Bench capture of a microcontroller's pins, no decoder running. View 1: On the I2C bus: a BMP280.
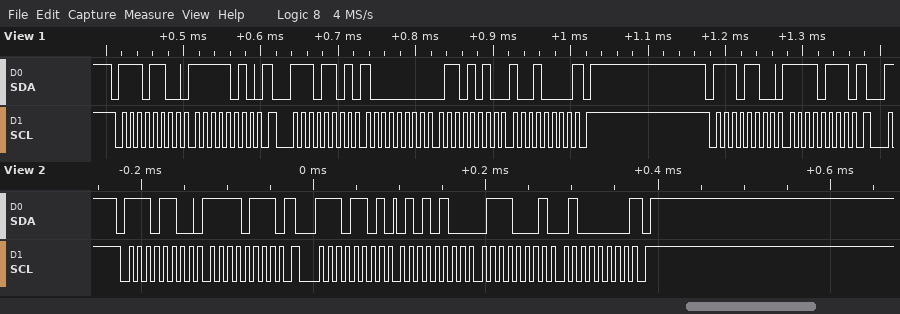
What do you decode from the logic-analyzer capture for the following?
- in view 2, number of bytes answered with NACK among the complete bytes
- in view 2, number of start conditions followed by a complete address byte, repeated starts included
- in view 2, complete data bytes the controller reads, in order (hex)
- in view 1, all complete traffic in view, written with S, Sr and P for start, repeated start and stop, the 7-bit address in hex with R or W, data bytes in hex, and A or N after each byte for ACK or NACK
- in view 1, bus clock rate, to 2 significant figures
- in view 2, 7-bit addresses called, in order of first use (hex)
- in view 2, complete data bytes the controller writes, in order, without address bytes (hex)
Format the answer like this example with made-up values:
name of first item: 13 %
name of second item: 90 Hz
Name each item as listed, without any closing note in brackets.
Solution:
in view 2, number of bytes answered with NACK among the complete bytes: 1
in view 2, number of start conditions followed by a complete address byte, repeated starts included: 2
in view 2, complete data bytes the controller reads, in order: 54 71 40
in view 1, all complete traffic in view, written with S, Sr and P for start, repeated start and stop, the 7-bit address in hex with R or W, data bytes in hex, and A or N after each byte for ACK or NACK: S 76W A FA A Sr 76R A 80 A 6A A 90 N P S 76W A F7 A
in view 1, bus clock rate, to 2 significant figures: 100 kHz
in view 2, 7-bit addresses called, in order of first use: 0x76
in view 2, complete data bytes the controller writes, in order, without address bytes: F7
